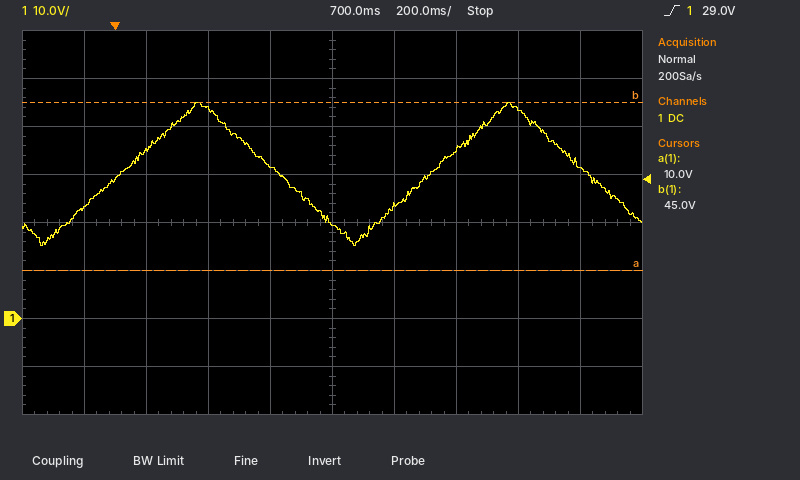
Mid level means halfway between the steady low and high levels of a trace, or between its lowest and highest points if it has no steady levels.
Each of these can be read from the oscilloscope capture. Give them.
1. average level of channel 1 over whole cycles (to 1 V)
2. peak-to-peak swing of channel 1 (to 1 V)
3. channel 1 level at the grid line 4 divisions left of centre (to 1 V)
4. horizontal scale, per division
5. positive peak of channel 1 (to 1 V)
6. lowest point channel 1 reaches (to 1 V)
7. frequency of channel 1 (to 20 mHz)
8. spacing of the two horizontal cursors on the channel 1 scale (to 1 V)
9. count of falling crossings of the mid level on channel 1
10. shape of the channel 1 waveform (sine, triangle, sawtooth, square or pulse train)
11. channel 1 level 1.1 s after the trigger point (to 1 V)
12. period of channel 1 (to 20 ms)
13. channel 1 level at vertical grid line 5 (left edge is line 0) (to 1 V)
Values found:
30 V
30 V
23 V
200 ms
45 V
15 V
1.00 Hz
35 V
2
triangle
35 V
1.00 s
20 V
